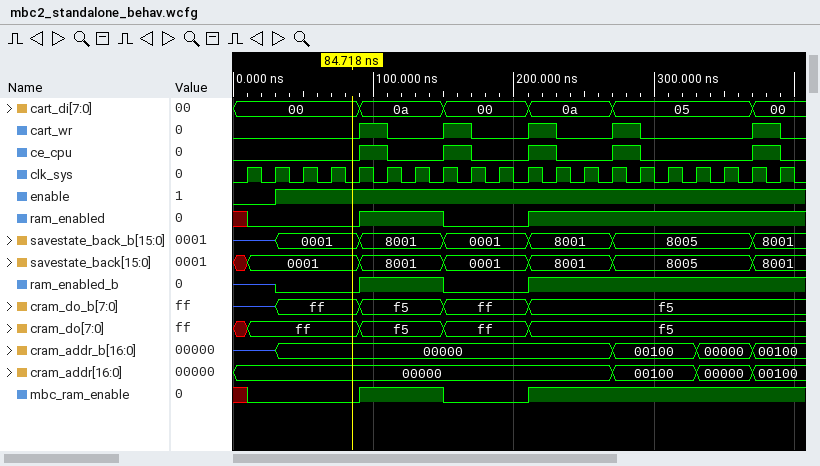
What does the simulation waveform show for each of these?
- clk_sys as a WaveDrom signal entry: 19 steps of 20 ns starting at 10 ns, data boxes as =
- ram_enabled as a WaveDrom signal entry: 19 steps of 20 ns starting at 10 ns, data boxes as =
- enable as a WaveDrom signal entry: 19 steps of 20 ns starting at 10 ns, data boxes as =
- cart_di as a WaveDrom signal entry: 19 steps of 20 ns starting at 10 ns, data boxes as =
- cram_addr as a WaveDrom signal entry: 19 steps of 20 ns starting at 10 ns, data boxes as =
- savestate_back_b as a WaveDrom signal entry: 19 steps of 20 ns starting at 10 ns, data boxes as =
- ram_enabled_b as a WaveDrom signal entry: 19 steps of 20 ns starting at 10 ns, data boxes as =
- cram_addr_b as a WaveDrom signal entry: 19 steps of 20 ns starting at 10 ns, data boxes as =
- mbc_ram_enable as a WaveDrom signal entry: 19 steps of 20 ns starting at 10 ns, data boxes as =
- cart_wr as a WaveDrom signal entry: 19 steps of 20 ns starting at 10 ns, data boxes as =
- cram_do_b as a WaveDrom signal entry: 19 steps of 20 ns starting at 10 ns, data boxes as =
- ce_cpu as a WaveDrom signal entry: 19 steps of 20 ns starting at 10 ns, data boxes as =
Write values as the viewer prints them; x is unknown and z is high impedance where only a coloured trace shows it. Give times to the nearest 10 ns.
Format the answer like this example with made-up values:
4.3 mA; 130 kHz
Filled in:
{name: 'clk_sys', wave: 'p..................'}; {name: 'ram_enabled', wave: '0...1..0..1........'}; {name: 'enable', wave: '01.................'}; {name: 'cart_di', wave: '=...=..=..=..=....=', data: '00 0a 00 0a 05 00'}; {name: 'cram_addr', wave: '=............=..=.=', data: '00000 00100 00000 00100'}; {name: 'savestate_back_b', wave: 'z=..=..=..=..=....=', data: '0001 8001 0001 8001 8005 8001'}; {name: 'ram_enabled_b', wave: 'z0..1..0..1........'}; {name: 'cram_addr_b', wave: 'z=...........=..=.=', data: '00000 00100 00000 00100'}; {name: 'mbc_ram_enable', wave: '0...1..0..1........'}; {name: 'cart_wr', wave: '0...10.10.10.10...1'}; {name: 'cram_do_b', wave: 'z=..=..=..=........', data: 'ff f5 ff f5'}; {name: 'ce_cpu', wave: '0...10.10.10.10...1'}
